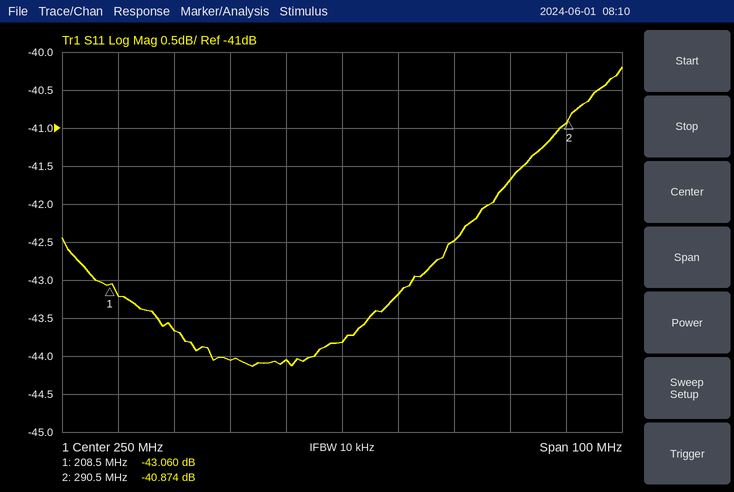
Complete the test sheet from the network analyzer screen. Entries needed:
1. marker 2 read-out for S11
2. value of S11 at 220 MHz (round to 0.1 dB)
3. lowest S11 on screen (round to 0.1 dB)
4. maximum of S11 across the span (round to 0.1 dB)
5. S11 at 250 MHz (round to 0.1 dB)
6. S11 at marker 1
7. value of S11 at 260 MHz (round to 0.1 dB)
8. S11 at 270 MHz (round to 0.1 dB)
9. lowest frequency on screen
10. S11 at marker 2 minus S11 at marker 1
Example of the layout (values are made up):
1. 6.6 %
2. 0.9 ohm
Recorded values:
1. -40.874 dB
2. -43.7 dB
3. -44.1 dB
4. -40.2 dB
5. -43.8 dB
6. -43.060 dB
7. -43.2 dB
8. -42.5 dB
9. 200 MHz
10. 2.186 dB
